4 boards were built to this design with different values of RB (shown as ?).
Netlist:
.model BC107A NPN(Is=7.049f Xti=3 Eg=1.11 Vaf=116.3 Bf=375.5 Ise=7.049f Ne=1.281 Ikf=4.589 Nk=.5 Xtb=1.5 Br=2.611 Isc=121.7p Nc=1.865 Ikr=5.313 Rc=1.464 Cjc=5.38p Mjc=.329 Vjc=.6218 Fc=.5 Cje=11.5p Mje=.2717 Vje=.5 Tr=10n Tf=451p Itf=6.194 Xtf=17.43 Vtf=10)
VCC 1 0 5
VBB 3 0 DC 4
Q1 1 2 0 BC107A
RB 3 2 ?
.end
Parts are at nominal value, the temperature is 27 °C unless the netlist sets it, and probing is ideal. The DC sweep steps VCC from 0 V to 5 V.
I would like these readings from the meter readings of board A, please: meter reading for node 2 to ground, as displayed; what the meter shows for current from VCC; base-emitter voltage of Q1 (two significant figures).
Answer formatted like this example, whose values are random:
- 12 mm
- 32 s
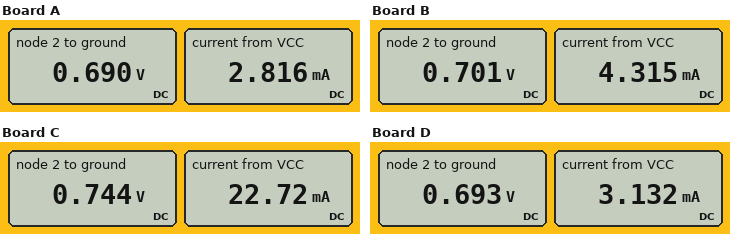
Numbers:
- 0.690 V
- 2.816 mA
- 690 mV
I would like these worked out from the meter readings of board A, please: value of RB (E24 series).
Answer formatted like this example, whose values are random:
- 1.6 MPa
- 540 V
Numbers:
- 220 kΩ
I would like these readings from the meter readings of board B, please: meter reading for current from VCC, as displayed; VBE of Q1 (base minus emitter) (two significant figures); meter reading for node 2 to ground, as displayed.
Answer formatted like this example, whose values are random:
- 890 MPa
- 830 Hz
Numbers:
- 4.315 mA
- 700 mV
- 0.701 V
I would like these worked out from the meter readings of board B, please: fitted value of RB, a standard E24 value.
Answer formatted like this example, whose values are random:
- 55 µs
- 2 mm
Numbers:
- 150 kΩ
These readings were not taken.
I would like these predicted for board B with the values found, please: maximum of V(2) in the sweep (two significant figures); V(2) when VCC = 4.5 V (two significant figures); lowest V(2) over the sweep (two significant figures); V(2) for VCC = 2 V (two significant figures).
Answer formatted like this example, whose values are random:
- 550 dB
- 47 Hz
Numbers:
- 700 mV
- 700 mV
- 560 mV
- 700 mV
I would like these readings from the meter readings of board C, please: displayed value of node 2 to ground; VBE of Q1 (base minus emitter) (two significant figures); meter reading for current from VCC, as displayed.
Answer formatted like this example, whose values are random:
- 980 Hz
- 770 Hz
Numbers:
- 0.744 V
- 740 mV
- 22.72 mA
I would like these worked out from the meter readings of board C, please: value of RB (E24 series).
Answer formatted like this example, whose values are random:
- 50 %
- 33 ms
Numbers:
- 33 kΩ
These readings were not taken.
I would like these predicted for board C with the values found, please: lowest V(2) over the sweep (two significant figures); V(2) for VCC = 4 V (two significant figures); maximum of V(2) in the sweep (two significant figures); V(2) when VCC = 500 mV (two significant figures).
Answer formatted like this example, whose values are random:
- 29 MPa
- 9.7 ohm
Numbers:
- 620 mV
- 740 mV
- 740 mV
- 740 mV
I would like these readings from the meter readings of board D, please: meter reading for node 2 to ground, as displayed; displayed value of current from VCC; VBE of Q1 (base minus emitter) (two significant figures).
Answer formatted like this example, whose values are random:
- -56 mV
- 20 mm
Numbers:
- 0.693 V
- 3.132 mA
- 690 mV
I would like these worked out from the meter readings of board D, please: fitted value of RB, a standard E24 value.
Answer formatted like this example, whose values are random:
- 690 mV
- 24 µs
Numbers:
- 200 kΩ
